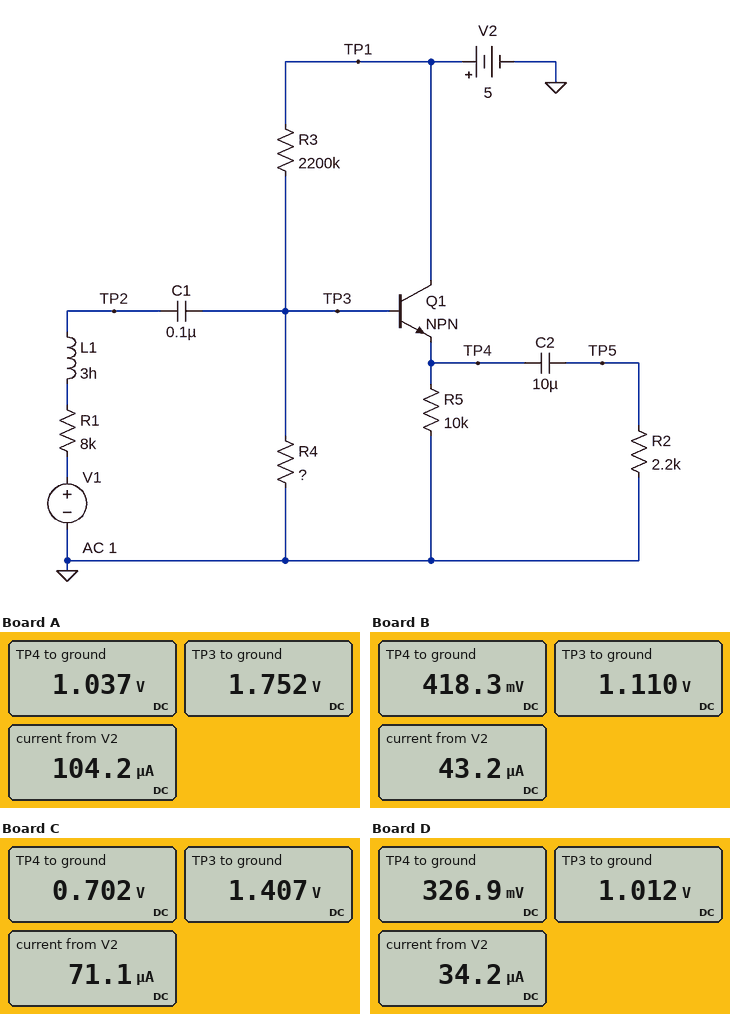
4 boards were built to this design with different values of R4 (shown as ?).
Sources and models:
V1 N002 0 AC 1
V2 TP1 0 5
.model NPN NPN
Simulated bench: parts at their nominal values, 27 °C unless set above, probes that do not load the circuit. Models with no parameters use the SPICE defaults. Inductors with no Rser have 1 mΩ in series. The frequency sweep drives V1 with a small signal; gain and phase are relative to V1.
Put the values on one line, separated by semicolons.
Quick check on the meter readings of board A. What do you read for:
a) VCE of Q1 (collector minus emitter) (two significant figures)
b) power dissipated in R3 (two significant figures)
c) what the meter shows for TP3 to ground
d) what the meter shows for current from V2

4.0 V; 4.8 µW; 1.752 V; 104.2 µA
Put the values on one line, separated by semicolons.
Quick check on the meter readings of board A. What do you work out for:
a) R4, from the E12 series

3.9 MΩ
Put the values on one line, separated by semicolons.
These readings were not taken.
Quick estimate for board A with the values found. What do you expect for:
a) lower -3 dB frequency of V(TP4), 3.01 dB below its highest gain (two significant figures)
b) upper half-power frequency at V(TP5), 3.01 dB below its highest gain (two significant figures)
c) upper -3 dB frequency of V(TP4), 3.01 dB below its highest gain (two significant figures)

9.1 Hz; 10 kHz; 10 kHz
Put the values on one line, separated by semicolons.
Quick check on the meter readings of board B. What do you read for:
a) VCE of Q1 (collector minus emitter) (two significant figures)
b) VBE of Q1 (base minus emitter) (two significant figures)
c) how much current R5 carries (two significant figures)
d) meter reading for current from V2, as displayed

4.6 V; 690 mV; 42 µA; 43.2 µA
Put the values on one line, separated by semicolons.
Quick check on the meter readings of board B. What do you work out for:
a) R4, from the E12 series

820 kΩ
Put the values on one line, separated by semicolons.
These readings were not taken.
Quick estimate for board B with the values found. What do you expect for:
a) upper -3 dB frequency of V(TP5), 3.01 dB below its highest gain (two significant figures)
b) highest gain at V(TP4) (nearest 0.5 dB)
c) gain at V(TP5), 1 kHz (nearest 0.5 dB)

9.6 kHz; -3.0 dB; -3.0 dB
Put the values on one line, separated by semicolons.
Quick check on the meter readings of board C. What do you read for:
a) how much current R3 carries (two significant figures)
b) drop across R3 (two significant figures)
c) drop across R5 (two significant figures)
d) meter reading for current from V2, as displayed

1.6 µA; 3.6 V; 700 mV; 71.1 µA
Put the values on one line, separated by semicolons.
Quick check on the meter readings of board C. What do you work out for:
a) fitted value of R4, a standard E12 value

1.5 MΩ
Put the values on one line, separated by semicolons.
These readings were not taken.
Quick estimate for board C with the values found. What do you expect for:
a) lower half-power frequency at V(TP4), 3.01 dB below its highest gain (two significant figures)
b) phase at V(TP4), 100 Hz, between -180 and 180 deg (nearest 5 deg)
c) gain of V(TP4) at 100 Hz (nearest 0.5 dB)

8.8 Hz; 5 deg; -2.0 dB
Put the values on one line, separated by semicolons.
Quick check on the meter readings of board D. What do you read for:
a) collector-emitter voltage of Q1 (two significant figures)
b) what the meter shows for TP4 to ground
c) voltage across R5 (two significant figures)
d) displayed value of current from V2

4.7 V; 326.9 mV; 330 mV; 34.2 µA
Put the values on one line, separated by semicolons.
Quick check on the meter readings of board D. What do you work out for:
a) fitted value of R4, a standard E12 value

680 kΩ
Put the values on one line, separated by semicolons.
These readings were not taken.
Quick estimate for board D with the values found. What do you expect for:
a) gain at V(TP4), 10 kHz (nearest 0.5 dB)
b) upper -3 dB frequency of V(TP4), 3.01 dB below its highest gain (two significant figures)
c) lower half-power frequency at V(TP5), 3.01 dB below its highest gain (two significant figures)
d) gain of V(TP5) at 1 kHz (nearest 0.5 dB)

-6.5 dB; 9.7 kHz; 12 Hz; -3.5 dB
